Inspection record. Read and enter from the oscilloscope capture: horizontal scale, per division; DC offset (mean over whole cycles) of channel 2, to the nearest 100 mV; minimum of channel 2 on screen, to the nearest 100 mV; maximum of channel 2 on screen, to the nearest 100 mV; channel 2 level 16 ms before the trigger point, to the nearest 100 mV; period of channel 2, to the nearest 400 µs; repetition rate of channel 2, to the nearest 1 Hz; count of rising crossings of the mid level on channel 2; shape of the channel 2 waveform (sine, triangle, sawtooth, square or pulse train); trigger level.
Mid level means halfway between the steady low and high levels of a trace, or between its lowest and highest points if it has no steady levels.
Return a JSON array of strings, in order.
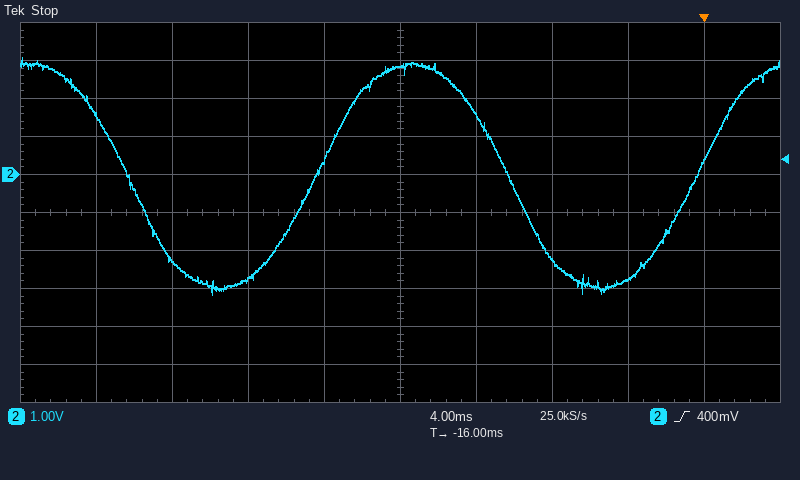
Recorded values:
["4 ms", "0.0 V", "-3.2 V", "3.1 V", "2.9 V", "20.0 ms", "50 Hz", "2", "sine", "400 mV"]
